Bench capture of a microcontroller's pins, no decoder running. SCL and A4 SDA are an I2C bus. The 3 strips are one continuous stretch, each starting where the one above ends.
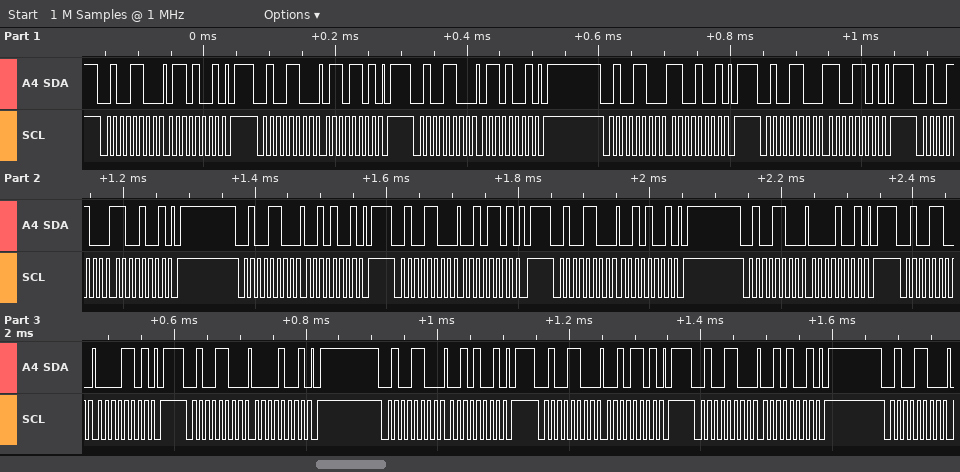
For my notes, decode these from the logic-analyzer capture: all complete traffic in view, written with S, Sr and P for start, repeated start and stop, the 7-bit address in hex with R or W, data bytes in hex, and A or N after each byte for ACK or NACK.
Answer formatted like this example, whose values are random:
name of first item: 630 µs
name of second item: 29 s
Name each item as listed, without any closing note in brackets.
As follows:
all complete traffic in view, written with S, Sr and P for start, repeated start and stop, the 7-bit address in hex with R or W, data bytes in hex, and A or N after each byte for ACK or NACK: S 26W A 69 A P S 26W A 6D A P S 26W A 69 A P S 26W A C9 A P S 26W A CD A P S 26W A C9 A P S 26W A 29 A P S 26W A 2D A P S 26W A 29 A P S 26W A 09 A P S 26W A 0D A P S 26W A 09 A P S 26W A 29 A P S 26W A 2D A P S 26W A 29 A P S 26W A
